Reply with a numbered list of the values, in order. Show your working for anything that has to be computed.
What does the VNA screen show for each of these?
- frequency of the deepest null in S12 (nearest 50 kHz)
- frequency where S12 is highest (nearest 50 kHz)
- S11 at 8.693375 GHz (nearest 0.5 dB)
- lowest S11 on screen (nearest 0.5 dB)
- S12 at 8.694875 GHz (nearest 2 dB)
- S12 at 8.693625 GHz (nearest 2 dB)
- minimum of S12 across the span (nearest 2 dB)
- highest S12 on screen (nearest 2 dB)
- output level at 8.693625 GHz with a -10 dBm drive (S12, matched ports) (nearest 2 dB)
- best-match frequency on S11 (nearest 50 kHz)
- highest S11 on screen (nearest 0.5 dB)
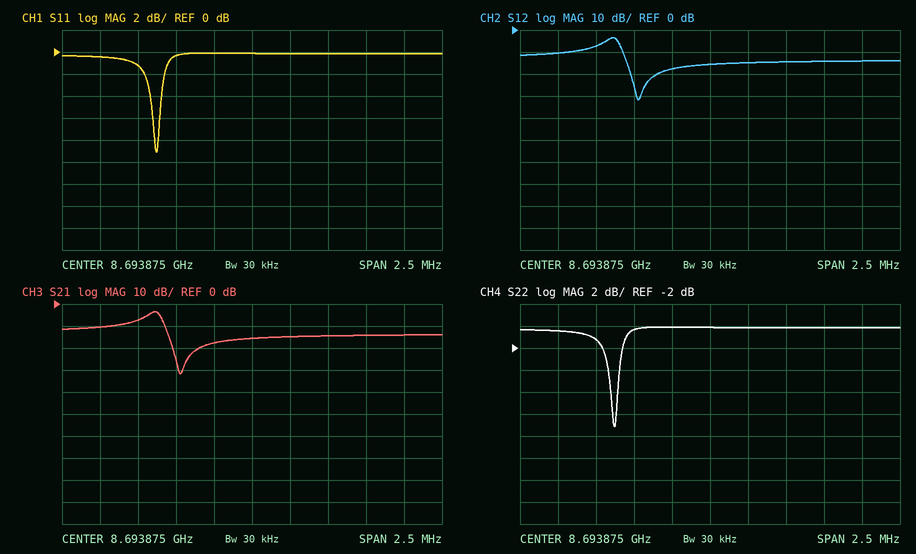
1. 8.69340 GHz
2. 8.69325 GHz
3. -0.5 dB
4. -9.0 dB
5. -14 dB
6. -18 dB
7. -32 dB
8. -4 dB
9. -10 dBm + (-18 dB) = -28 dBm
10. 8.69325 GHz
11. 0.0 dB
